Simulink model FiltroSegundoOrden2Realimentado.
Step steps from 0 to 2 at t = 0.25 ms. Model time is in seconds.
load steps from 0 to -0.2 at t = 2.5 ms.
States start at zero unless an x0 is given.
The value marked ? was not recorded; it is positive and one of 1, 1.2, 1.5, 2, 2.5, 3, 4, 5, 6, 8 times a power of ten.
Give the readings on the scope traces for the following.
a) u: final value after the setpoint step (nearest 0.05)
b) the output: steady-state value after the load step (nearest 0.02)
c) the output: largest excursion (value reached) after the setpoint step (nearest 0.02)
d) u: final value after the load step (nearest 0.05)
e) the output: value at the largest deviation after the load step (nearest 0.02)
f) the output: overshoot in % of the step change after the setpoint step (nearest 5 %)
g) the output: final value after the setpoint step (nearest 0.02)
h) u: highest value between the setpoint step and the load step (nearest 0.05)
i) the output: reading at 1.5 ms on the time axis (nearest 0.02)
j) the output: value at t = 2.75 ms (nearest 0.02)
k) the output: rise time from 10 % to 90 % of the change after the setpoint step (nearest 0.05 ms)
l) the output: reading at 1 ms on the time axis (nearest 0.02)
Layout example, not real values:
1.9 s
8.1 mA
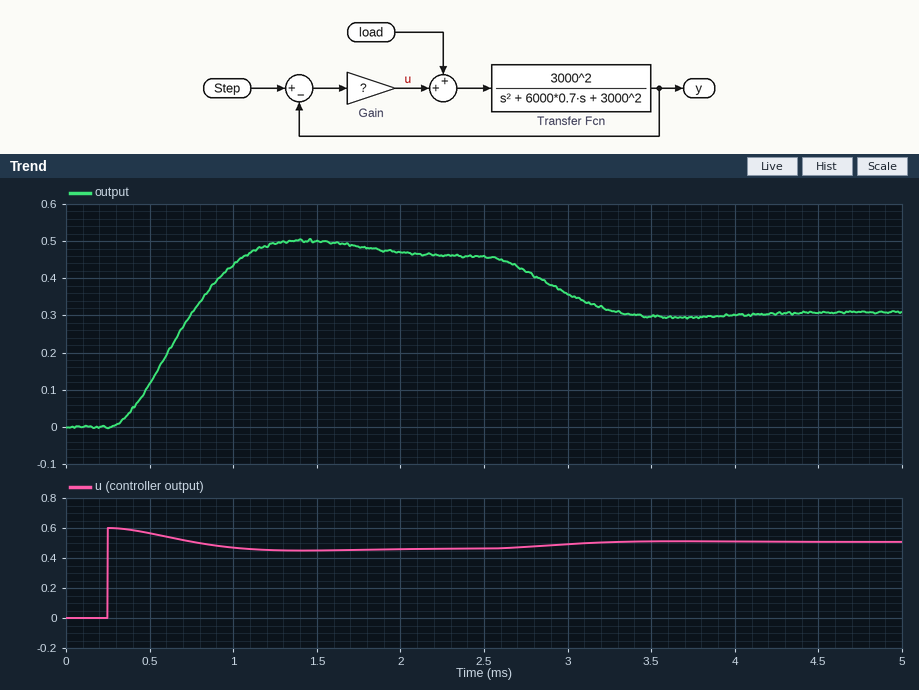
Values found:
0.45
0.30
0.50
0.50
0.30
10 %
0.46
0.60
0.50
0.42
0.55 ms
0.44
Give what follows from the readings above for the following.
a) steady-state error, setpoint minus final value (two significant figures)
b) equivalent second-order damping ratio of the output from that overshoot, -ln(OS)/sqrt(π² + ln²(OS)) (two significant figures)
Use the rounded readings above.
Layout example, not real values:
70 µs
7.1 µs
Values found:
1.5
0.59
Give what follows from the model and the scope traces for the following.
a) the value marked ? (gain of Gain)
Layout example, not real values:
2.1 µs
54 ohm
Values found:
0.3
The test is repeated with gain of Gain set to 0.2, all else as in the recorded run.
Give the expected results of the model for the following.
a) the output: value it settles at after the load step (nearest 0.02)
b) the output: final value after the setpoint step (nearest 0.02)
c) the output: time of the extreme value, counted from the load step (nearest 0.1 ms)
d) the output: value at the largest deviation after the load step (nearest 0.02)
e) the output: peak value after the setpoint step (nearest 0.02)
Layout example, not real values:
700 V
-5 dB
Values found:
0.16
0.34
1.2 ms
0.16
0.36
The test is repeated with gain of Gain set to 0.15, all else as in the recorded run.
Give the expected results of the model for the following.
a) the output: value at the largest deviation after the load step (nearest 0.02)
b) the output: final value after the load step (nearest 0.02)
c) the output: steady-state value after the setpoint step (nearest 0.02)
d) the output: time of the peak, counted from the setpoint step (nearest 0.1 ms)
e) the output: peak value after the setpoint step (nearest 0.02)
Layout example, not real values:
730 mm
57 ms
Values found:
0.08
0.08
0.26
1.3 ms
0.28
